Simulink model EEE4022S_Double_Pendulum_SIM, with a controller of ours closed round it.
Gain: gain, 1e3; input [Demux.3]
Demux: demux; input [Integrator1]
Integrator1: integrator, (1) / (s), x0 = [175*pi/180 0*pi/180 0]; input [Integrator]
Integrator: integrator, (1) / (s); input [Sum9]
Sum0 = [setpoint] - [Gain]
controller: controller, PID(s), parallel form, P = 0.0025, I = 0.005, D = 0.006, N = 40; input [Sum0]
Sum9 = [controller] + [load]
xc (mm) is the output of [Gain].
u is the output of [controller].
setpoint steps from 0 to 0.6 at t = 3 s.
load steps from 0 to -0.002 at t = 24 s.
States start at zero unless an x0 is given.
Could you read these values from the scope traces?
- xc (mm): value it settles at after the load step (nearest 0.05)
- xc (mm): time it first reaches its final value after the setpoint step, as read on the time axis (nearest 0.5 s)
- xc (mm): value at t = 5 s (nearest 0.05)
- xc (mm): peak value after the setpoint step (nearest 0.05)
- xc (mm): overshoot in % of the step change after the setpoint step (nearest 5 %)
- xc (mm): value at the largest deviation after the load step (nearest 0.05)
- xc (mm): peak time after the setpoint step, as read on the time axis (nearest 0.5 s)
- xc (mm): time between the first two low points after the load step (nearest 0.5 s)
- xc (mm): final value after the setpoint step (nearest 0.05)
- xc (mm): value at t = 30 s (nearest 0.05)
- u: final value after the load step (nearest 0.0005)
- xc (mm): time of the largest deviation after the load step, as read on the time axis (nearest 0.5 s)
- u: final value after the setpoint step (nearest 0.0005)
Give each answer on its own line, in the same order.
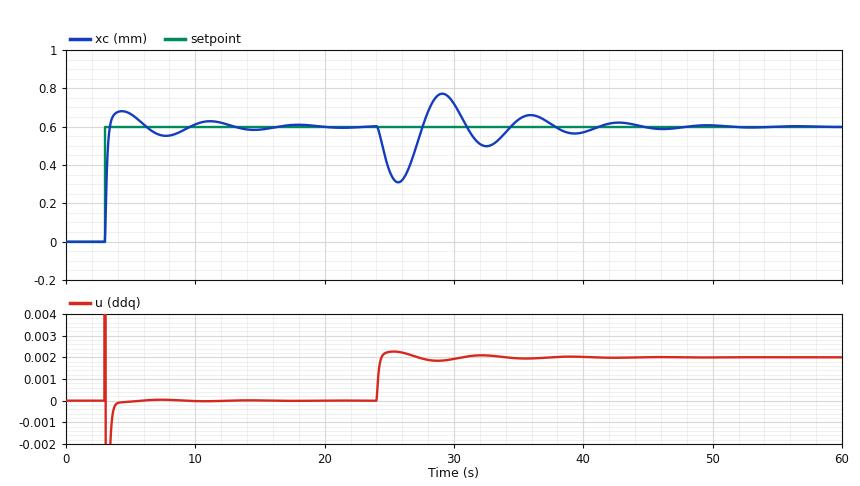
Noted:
0.60
3.5 s
0.65
0.70
15 %
0.30
4.5 s
7.0 s
0.60
0.70
0.0020
25.5 s
0.0000
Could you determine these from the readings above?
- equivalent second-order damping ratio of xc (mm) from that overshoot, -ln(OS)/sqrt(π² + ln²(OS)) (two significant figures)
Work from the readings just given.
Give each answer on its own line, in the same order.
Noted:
0.52
